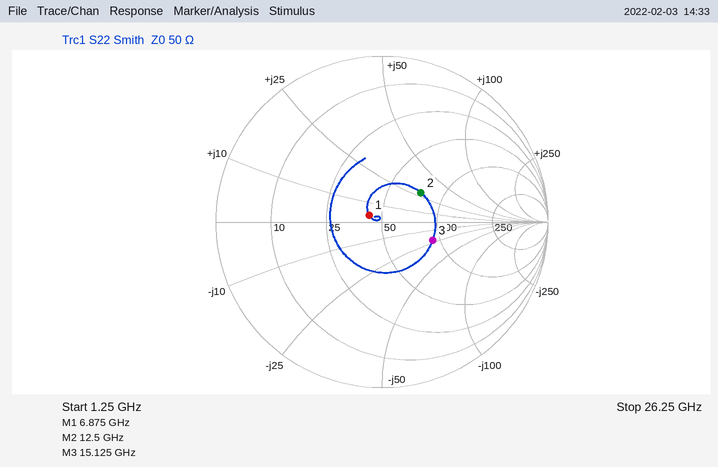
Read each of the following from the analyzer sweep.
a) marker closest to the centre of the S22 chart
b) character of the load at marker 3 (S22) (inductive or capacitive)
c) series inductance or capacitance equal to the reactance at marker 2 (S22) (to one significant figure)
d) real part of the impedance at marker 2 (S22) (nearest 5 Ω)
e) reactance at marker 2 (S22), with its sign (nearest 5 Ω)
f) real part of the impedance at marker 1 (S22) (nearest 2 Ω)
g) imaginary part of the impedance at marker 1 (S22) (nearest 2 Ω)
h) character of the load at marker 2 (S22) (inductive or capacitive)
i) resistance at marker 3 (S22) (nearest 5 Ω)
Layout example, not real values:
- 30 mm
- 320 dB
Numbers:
- marker 1
- capacitive
- 400 pH
- 75 Ω
- +30 Ω
- 42 Ω
- +4 Ω
- inductive
- 90 Ω
